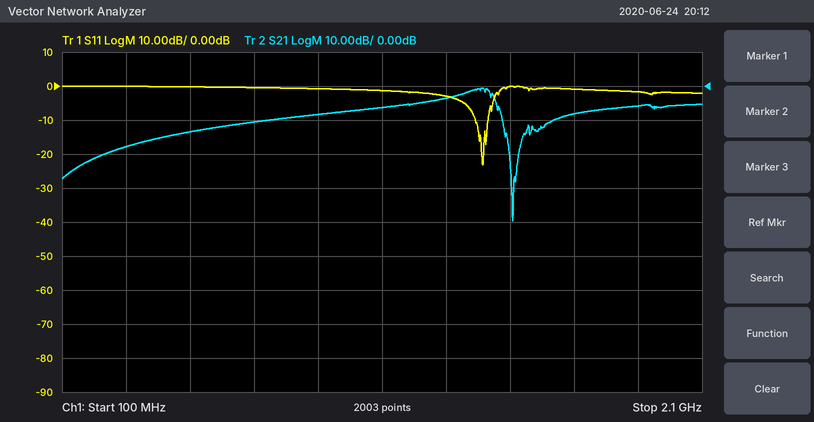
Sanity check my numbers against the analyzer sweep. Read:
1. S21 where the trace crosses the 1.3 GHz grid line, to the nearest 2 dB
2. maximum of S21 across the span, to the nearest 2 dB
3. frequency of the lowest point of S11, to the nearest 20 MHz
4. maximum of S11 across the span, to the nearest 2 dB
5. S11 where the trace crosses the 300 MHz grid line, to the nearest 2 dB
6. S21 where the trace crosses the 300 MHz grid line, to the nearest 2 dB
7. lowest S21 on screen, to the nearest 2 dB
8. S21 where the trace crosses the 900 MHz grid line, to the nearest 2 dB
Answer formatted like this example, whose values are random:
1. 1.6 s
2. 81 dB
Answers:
1. -4 dB
2. 0 dB
3. 1.42 GHz
4. 0 dB
5. 0 dB
6. -18 dB
7. -40 dB
8. -8 dB
